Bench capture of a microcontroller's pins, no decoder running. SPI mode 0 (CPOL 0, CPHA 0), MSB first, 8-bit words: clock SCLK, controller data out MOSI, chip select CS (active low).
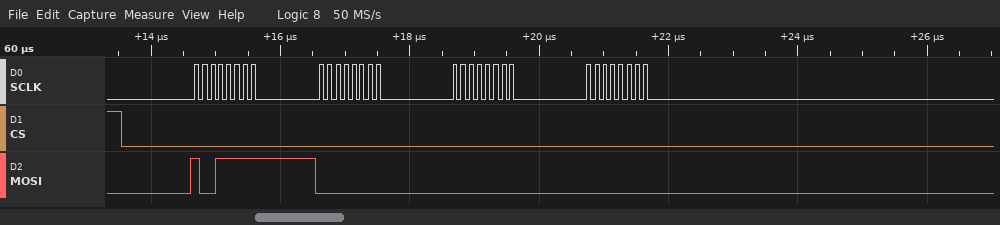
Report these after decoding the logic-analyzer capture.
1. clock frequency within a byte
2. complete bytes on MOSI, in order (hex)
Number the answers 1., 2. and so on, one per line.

1. 8 MHz
2. 9F 00 00 00
